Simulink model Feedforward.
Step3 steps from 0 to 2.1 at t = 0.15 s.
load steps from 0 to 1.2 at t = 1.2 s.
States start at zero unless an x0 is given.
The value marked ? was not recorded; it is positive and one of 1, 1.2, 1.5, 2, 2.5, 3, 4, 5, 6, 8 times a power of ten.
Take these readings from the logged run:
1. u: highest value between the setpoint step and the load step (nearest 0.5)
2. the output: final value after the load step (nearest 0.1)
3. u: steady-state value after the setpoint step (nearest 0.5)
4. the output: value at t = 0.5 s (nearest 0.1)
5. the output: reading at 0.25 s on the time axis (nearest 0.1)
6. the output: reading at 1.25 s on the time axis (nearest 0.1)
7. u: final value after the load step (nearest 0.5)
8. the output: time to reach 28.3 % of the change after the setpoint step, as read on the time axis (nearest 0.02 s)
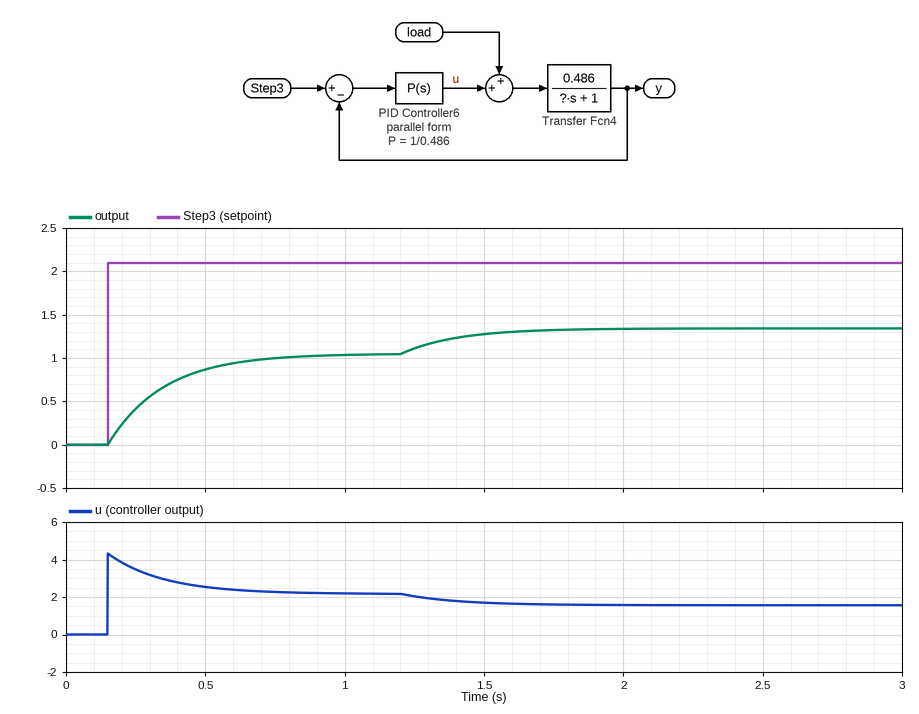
4.5
1.3
2.0
0.9
0.4
1.1
1.5
0.22 s
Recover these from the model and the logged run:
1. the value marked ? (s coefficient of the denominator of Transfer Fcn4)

0.4
